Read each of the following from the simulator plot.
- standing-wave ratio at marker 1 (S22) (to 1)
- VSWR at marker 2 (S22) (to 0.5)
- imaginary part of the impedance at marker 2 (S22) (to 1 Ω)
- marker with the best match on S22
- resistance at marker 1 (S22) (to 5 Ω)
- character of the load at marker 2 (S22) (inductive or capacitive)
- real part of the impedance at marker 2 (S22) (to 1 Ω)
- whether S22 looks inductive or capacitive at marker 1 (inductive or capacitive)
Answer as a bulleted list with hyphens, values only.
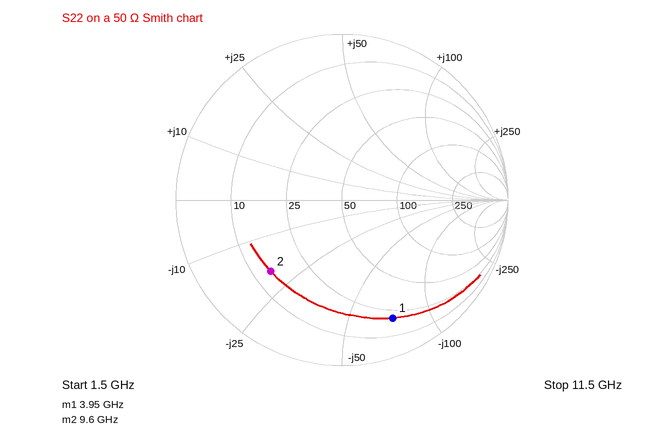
- 8
- 4.0
- -19 Ω
- marker 2
- 20 Ω
- capacitive
- 14 Ω
- capacitive
